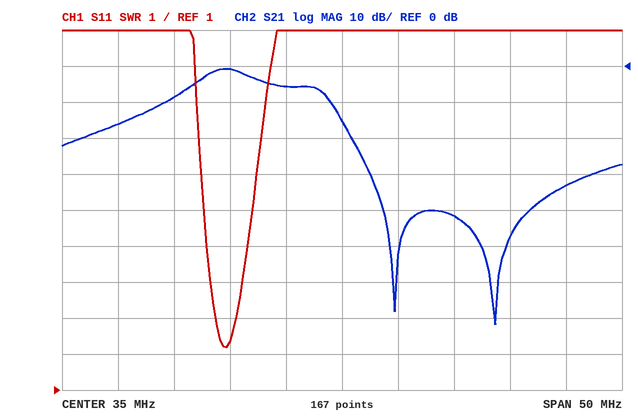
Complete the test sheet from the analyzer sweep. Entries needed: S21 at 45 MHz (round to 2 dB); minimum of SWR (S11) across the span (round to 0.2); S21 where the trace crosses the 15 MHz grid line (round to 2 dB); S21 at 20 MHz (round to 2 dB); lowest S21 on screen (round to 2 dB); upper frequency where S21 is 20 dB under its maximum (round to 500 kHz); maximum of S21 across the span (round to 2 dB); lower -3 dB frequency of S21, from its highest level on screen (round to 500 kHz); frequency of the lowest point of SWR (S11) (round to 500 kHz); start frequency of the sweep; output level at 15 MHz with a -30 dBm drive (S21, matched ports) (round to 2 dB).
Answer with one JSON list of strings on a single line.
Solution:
["-42 dB", "2.2", "-16 dB", "-8 dB", "-72 dB", "36.0 MHz", "0 dB", "22.5 MHz", "24.5 MHz", "10 MHz", "-46 dBm"]
